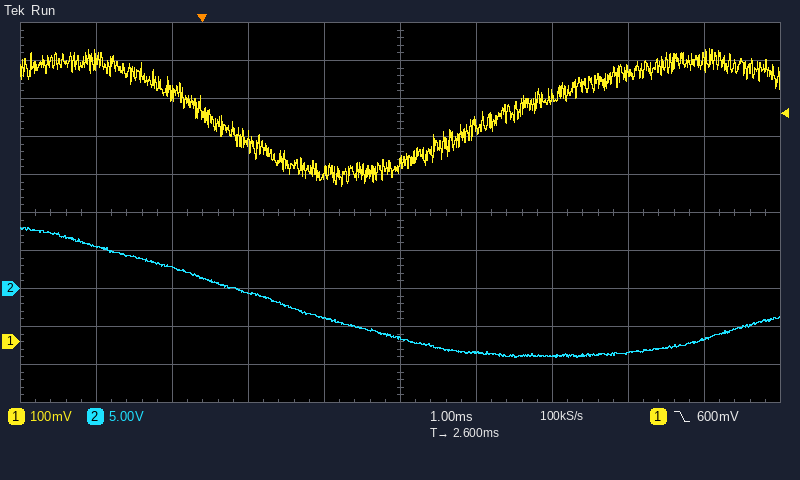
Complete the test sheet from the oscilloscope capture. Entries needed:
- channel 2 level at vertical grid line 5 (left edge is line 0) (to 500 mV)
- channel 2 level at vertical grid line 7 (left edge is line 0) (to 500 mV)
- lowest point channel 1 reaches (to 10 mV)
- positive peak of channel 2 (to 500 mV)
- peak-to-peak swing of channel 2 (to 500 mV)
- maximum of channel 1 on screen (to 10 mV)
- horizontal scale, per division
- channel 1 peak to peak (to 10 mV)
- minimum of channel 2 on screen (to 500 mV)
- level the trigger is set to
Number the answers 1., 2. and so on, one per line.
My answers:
1. -6.5 V
2. -9.0 V
3. 410 mV
4. 8.0 V
5. 17.0 V
6. 770 mV
7. 1 ms
8. 360 mV
9. -9.0 V
10. 600 mV
